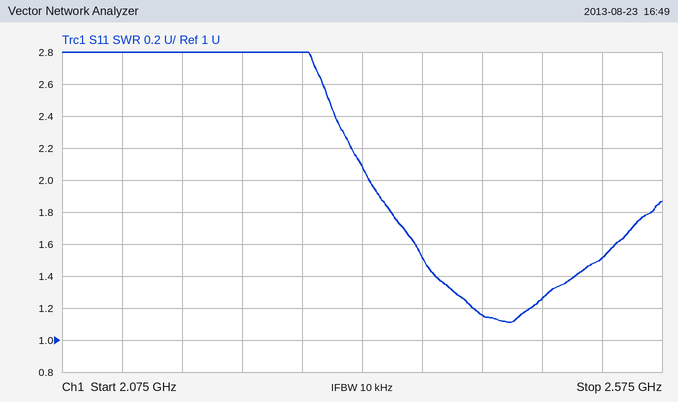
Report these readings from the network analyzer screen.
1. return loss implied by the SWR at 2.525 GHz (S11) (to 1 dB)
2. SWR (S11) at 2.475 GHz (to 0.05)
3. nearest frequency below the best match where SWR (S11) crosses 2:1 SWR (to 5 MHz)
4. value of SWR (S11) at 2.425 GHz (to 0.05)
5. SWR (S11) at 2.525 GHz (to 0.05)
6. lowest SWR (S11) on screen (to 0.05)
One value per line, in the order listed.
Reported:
14 dB
1.25
2.330 GHz
1.15
1.50
1.10
